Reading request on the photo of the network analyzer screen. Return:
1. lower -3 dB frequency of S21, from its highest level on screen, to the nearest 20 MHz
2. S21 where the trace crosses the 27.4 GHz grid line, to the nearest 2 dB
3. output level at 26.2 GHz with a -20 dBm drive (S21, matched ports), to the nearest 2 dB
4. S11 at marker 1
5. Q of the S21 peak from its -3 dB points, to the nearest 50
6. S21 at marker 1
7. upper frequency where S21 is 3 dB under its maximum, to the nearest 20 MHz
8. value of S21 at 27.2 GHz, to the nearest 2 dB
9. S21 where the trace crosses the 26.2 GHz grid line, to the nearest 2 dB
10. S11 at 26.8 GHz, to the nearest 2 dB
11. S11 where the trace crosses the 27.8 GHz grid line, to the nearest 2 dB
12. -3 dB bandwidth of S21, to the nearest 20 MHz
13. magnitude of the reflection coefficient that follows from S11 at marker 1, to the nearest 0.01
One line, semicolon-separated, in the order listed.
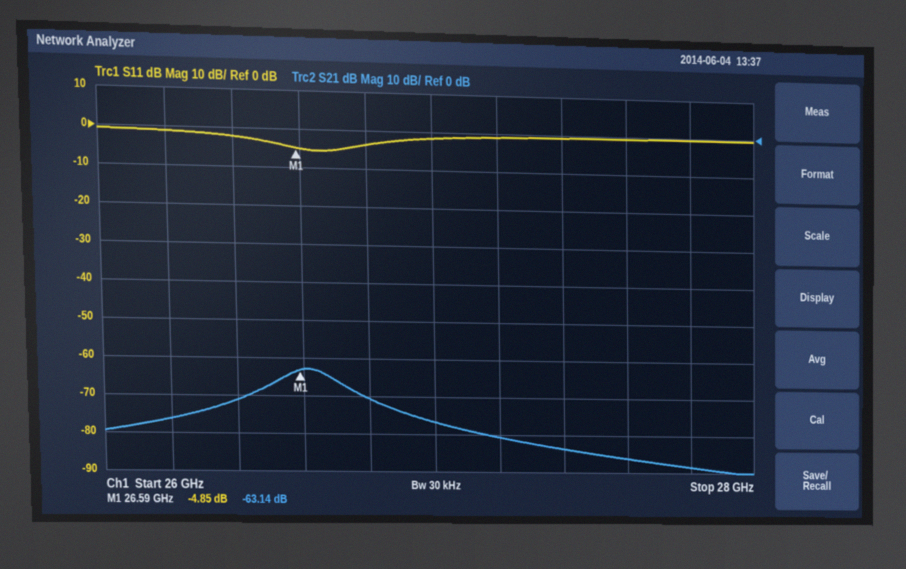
26.52 GHz; -84 dB; -96 dBm; -4.85 dB; 150; -63.14 dB; 26.70 GHz; -80 dB; -76 dB; -4 dB; 0 dB; 180 MHz; 0.57
